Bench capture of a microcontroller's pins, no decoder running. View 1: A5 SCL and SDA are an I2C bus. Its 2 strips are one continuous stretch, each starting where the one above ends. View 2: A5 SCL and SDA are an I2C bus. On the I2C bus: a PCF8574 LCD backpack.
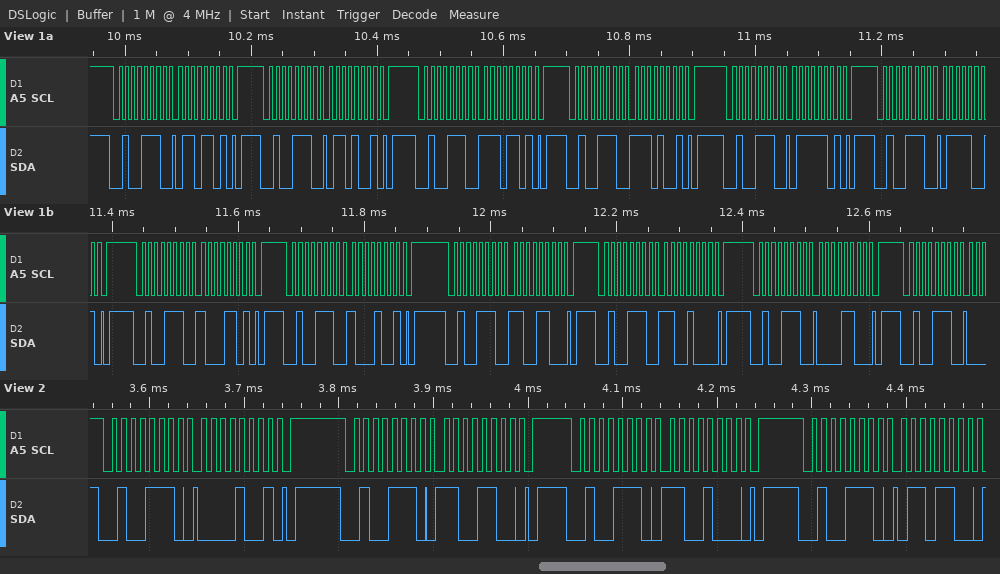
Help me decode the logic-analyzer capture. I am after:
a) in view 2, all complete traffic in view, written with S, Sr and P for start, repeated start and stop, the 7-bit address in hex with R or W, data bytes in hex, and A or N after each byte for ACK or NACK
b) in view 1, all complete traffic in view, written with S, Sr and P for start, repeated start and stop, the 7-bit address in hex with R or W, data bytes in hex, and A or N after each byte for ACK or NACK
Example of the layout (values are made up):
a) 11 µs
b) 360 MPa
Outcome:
a) S 27W A 09 A P S 27W A CC A P S 27W A C8 A P S 27W A 6C A
b) S 27W A 6D A P S 27W A 69 A P S 27W A ED A P S 27W A E9 A P S 27W A 7D A P S 27W A 79 A P S 27W A 8D A P S 27W A 89 A P S 27W A CC A P S 27W A C8 A P S 27W A 0C A P S 27W A
